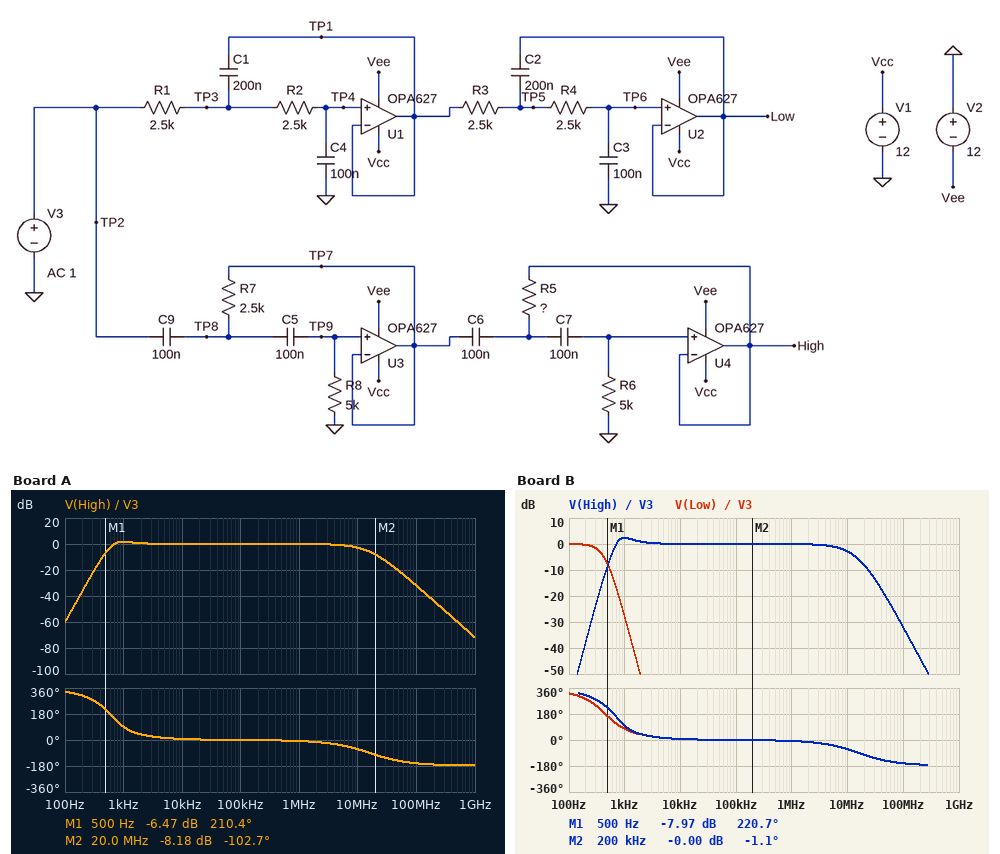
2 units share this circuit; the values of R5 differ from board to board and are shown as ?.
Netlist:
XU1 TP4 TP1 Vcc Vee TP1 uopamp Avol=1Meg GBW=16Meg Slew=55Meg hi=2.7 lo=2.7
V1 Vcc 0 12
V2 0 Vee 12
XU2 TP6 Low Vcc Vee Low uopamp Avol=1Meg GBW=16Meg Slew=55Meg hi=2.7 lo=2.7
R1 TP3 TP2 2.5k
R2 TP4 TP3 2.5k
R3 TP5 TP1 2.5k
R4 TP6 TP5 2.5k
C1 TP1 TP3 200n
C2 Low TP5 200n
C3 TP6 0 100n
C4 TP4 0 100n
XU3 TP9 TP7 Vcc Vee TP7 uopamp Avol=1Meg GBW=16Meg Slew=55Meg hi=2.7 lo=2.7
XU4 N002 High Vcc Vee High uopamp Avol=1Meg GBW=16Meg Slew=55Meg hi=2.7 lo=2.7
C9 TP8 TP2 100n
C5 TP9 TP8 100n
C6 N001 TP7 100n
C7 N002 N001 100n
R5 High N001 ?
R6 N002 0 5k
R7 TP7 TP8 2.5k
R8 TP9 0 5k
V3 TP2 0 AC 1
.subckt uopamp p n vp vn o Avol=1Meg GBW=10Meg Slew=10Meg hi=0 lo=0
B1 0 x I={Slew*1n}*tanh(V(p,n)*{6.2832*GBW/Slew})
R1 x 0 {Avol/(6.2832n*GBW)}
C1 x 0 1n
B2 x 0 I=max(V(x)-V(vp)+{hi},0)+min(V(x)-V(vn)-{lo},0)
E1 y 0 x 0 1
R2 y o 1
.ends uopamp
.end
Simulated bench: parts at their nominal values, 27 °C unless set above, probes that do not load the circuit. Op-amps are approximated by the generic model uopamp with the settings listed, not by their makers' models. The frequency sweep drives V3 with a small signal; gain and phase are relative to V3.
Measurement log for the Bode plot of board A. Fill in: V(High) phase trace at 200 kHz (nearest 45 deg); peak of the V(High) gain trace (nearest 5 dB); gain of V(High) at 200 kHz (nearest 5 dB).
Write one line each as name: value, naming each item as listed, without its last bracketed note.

V(High) phase trace at 200 kHz: 0 deg
peak of the V(High) gain trace: 0 dB
gain of V(High) at 200 kHz: 0 dB
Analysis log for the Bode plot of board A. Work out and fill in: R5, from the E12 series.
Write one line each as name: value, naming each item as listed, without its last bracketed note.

R5, from the E12 series: 1 kΩ
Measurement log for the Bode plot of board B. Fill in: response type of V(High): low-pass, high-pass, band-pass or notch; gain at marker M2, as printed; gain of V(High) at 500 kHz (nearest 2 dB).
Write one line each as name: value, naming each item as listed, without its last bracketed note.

response type of V(High): low-pass, high-pass, band-pass or notch: band-pass
gain at marker M2, as printed: -0.00 dB
gain of V(High) at 500 kHz: 0 dB
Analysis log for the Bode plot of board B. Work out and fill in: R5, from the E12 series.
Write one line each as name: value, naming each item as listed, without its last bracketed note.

R5, from the E12 series: 820 Ω
